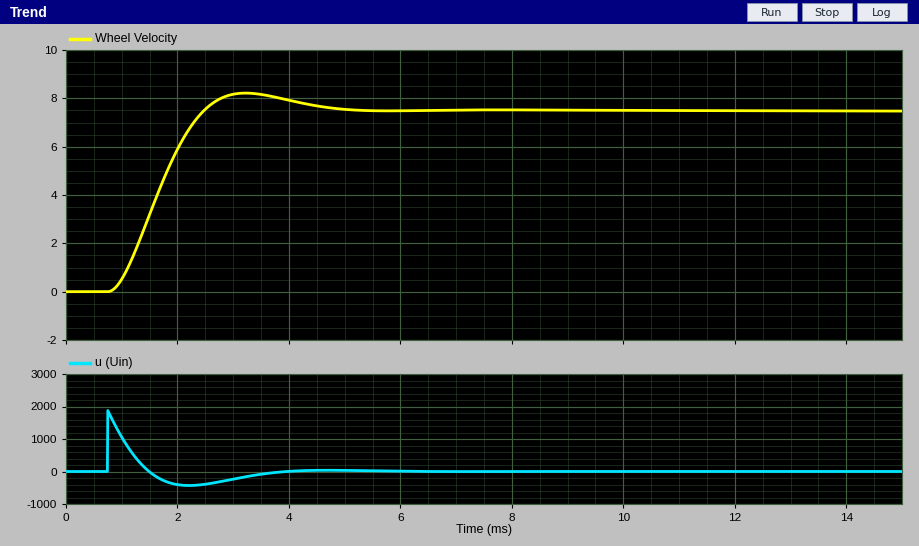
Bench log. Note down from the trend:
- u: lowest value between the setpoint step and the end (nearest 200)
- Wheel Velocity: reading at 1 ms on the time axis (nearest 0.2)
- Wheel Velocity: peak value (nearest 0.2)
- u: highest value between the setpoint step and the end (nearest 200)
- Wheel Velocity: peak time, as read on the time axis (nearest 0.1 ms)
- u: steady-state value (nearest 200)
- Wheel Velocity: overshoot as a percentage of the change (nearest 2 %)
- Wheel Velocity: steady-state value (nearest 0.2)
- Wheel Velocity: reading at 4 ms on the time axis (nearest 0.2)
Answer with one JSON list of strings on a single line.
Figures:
["-400", "0.6", "8.2", "1800", "3.2 ms", "0", "10 %", "7.4", "8.0"]
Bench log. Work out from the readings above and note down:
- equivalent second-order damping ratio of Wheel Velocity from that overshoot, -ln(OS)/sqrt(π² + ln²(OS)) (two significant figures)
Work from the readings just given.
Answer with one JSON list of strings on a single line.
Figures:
["0.59"]
